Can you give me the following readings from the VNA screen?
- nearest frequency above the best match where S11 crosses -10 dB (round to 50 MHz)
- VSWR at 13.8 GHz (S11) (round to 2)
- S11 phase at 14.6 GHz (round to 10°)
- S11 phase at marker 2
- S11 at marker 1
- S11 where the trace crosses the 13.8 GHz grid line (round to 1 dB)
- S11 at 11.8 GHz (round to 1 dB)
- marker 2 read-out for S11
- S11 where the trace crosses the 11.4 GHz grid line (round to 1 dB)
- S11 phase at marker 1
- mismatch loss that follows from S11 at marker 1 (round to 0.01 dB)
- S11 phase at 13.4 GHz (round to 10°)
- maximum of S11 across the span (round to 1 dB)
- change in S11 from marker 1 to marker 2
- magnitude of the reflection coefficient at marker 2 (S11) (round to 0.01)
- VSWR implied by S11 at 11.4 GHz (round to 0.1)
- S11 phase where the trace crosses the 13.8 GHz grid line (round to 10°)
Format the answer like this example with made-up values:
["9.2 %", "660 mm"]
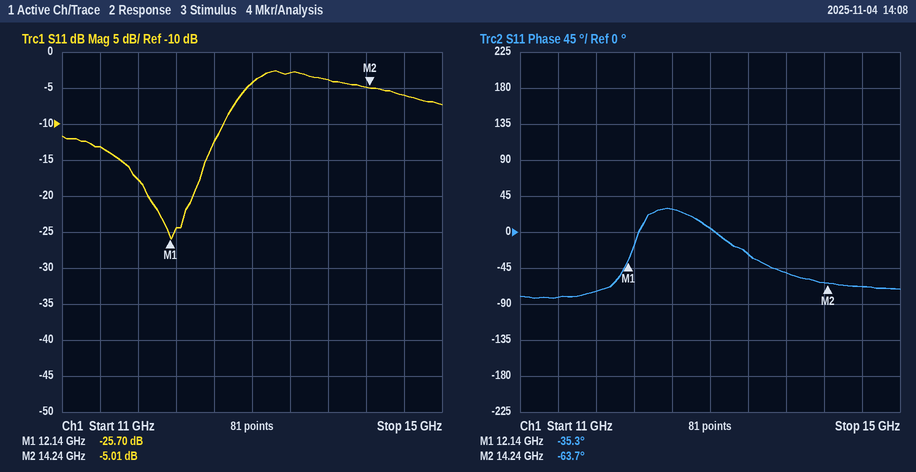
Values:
["12.70 GHz", "4", "-70°", "-63.7°", "-25.70 dB", "-4 dB", "-18 dB", "-5.01 dB", "-13 dB", "-35.3°", "0.01 dB", "-30°", "-3 dB", "20.69 dB", "0.56", "1.6", "-50°"]
